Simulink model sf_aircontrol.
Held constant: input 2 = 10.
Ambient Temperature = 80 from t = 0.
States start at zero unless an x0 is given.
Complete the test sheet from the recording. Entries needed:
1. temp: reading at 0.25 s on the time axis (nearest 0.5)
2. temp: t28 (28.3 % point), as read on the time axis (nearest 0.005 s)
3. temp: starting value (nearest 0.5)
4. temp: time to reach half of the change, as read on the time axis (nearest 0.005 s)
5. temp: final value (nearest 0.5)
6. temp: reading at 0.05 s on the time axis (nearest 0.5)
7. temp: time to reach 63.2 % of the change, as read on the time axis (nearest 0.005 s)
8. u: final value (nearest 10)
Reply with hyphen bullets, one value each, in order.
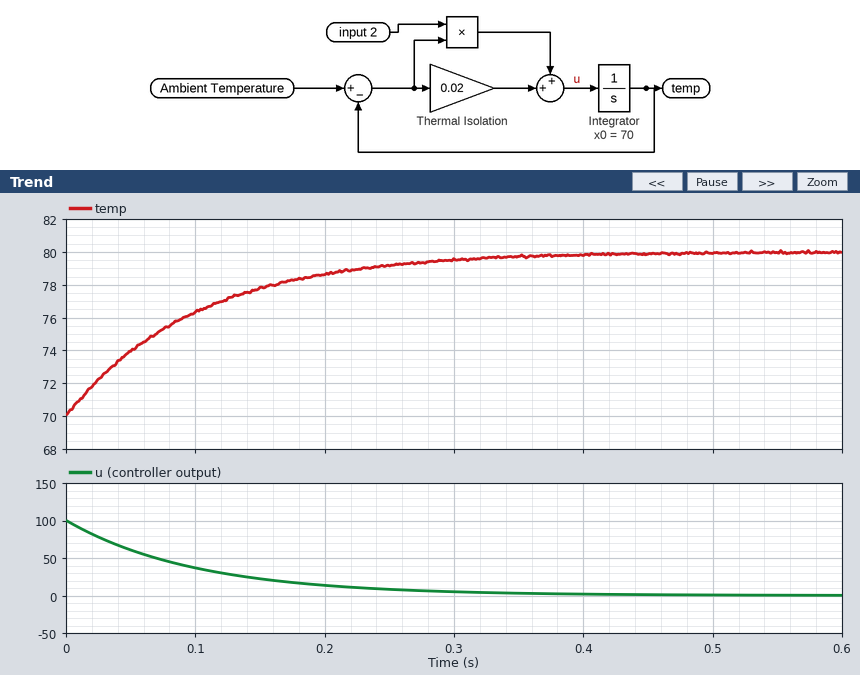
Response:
- 79.0
- 0.035 s
- 70.0
- 0.070 s
- 80.0
- 74.0
- 0.100 s
- 0
